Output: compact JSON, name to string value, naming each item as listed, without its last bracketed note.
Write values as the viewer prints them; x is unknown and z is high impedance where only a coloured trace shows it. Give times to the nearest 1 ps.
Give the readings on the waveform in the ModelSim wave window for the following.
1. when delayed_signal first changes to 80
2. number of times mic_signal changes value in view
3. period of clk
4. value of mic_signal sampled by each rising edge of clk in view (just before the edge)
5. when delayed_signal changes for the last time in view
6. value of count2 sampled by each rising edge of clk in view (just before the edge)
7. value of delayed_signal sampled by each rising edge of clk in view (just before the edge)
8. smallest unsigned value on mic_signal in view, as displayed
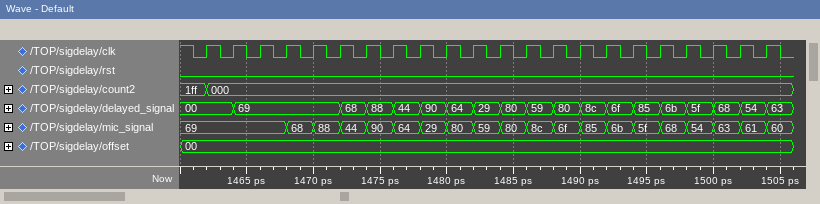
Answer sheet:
{"when delayed_signal first changes to 80": "1484 ps", "number of times mic_signal changes value in view": "19", "period of clk": "2 ps", "value of mic_signal sampled by each rising edge of clk in view": "69, 69, 69, 69, 68, 88, 44, 90, 64, 29, 80, 59, 80, 8c, 6f, 85, 6b, 5f, 68, 54, 63, 61", "when delayed_signal changes for the last time in view": "1504 ps", "value of count2 sampled by each rising edge of clk in view": "1ff, 000, 000, 000, 000, 000, 000, 000, 000, 000, 000, 000, 000, 000, 000, 000, 000, 000, 000, 000, 000, 000", "value of delayed_signal sampled by each rising edge of clk in view": "00, 00, 69, 69, 69, 69, 68, 88, 44, 90, 64, 29, 80, 59, 80, 8c, 6f, 85, 6b, 5f, 68, 54", "smallest unsigned value on mic_signal in view, as displayed": "29"}
